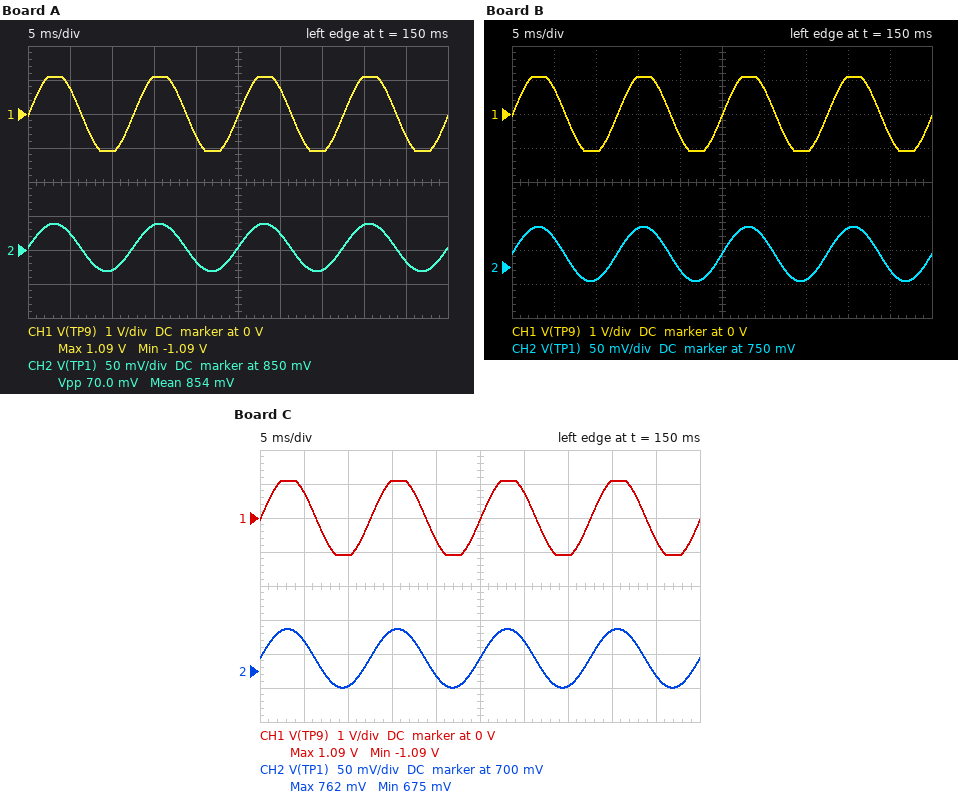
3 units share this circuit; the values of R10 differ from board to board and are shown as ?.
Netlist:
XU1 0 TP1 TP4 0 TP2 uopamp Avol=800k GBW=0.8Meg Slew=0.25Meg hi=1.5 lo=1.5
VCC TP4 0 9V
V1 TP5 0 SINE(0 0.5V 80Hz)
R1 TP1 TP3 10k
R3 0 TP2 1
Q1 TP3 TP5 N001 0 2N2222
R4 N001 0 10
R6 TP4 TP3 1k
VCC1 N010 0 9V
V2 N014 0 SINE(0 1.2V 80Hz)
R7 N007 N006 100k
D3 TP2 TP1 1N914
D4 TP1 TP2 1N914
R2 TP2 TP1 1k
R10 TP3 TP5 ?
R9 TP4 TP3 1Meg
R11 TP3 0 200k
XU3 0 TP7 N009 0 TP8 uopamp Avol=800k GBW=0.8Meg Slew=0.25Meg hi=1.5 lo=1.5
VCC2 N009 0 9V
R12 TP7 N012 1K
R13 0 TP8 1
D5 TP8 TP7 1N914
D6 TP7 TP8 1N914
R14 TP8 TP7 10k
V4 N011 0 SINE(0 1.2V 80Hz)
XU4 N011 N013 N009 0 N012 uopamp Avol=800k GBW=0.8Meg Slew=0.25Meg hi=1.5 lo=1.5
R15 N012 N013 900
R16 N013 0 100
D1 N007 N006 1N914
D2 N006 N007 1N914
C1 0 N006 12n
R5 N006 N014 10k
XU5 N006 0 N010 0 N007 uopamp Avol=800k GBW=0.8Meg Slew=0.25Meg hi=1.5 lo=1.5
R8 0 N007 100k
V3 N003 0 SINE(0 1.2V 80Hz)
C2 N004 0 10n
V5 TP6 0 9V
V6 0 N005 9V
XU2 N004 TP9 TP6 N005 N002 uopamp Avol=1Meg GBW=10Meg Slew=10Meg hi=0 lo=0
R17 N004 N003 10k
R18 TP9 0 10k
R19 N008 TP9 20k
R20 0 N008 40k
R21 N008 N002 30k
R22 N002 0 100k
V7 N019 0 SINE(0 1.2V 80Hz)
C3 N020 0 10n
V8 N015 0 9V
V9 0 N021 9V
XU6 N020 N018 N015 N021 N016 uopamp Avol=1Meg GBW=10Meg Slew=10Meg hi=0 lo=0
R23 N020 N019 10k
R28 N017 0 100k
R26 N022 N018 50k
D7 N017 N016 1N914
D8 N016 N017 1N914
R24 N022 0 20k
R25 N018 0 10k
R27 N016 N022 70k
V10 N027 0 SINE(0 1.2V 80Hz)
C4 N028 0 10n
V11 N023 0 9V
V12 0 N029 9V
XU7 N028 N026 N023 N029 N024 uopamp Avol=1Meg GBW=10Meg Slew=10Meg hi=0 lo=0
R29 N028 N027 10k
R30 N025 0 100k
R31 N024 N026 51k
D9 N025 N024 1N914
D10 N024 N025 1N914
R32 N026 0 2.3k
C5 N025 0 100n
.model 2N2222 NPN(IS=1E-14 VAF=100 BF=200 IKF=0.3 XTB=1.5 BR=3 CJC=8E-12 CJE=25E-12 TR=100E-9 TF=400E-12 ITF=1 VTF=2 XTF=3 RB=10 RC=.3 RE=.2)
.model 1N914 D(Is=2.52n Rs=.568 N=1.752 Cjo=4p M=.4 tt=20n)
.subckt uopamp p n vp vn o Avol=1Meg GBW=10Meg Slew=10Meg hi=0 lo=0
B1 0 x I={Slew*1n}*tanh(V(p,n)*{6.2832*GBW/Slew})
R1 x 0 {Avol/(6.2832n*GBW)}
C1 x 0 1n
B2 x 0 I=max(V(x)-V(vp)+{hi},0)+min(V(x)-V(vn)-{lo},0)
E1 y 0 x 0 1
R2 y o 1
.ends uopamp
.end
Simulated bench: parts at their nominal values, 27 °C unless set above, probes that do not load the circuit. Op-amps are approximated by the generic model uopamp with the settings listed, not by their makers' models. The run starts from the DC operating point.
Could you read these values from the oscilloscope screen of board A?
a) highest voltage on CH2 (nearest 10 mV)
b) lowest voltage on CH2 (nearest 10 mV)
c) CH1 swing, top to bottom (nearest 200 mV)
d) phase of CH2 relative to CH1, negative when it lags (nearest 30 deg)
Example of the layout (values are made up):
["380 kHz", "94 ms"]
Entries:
["890 mV", "820 mV", "2.2 V", "0 deg"]
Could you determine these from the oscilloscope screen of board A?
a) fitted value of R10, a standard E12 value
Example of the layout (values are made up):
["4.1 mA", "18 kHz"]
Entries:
["270 Ω"]
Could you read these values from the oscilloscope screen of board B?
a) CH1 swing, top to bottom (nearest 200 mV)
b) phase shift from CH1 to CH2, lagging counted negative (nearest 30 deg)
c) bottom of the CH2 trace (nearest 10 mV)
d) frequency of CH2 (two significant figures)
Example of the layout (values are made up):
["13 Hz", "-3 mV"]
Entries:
["2.2 V", "0 deg", "730 mV", "80 Hz"]
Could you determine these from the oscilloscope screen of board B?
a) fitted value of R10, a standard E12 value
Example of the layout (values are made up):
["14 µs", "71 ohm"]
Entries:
["120 Ω"]
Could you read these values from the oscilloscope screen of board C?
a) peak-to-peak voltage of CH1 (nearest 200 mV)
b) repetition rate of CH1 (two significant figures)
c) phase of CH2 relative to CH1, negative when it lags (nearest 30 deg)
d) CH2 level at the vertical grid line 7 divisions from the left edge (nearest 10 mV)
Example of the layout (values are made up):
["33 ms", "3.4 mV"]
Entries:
["2.2 V", "80 Hz", "0 deg", "680 mV"]
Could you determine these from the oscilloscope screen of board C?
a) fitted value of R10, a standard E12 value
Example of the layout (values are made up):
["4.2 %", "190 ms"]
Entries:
["47 Ω"]
